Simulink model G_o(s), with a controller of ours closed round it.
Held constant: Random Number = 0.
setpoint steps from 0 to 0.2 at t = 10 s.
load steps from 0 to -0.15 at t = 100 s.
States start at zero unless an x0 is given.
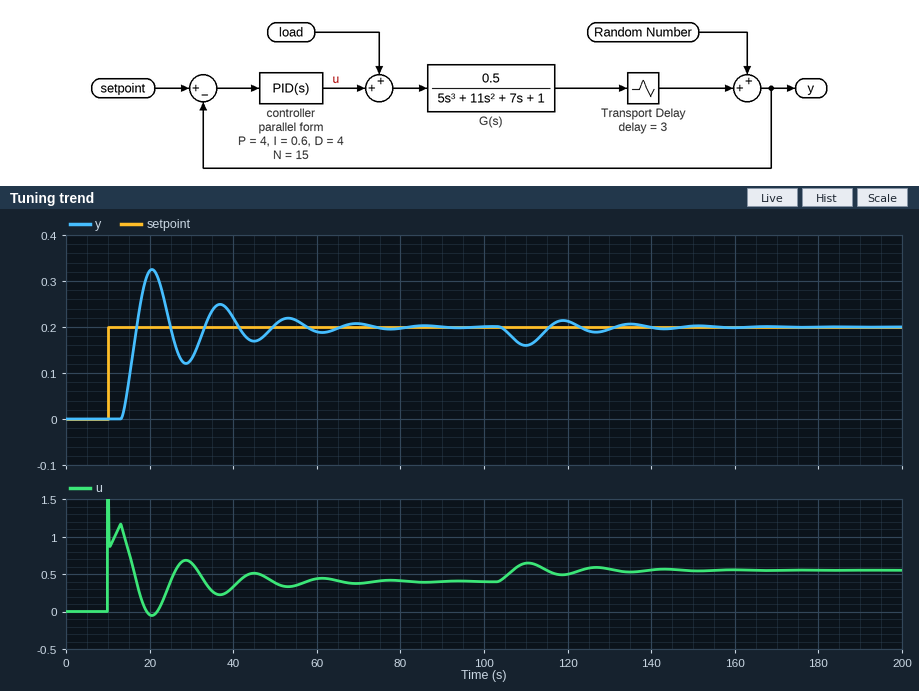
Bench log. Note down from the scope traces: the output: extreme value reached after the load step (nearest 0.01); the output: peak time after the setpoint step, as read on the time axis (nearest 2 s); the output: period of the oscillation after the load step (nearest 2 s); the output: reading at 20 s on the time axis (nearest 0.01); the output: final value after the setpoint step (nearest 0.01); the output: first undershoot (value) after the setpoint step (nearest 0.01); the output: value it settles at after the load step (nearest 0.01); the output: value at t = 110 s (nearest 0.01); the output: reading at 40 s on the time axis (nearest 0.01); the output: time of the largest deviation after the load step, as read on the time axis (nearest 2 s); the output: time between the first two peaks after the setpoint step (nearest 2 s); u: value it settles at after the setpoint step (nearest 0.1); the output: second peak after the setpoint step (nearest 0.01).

0.16
20 s
16 s
0.32
0.20
0.12
0.20
0.16
0.22
110 s
16 s
0.4
0.25
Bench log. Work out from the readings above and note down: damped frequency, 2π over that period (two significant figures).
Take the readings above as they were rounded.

0.39 rad/s
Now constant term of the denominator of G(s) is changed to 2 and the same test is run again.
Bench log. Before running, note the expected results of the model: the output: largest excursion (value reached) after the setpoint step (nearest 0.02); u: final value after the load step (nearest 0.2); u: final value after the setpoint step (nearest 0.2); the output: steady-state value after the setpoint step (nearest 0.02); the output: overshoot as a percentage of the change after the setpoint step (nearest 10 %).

0.24
1.0
0.8
0.20
20 %
